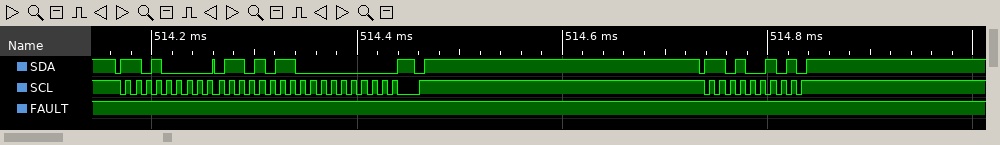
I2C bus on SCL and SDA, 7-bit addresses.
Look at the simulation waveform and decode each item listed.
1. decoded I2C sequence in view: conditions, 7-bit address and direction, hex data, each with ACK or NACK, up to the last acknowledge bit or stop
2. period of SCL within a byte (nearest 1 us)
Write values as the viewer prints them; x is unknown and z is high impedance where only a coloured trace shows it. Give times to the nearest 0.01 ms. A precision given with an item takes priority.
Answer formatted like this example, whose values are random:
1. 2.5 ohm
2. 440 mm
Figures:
1. start, address 68 write ACK, 6B ACK, 00 ACK, stop, start, address 69 write NACK, stop
2. 10 us
